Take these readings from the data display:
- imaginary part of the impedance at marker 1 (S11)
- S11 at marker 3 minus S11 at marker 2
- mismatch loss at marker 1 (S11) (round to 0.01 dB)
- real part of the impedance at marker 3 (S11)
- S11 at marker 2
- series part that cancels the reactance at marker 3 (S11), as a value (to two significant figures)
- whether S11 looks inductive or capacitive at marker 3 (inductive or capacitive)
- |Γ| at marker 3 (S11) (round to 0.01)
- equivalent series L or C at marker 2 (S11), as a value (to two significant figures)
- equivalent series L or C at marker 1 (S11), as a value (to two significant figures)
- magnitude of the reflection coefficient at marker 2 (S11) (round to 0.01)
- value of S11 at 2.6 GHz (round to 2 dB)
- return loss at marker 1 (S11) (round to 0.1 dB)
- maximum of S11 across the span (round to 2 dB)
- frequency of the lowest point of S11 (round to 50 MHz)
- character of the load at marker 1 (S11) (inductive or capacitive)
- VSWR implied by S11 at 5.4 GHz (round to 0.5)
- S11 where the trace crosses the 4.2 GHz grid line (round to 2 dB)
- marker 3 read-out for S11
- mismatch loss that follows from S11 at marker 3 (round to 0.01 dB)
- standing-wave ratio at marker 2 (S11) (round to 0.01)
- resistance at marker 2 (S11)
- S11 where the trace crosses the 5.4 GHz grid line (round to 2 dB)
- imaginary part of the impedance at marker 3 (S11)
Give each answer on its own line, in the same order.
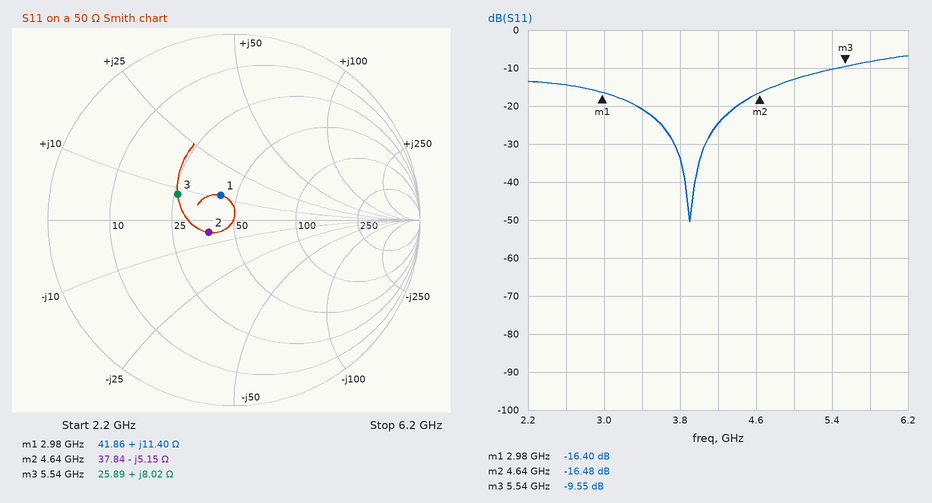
+11.40 Ω
6.93 dB
0.10 dB
25.89 Ω
-16.48 dB
3.6 pF
inductive
0.33
6.7 pF
610 pH
0.15
-14 dB
16.4 dB
-6 dB
3.90 GHz
inductive
2.0
-24 dB
-9.55 dB
0.51 dB
1.35
37.84 Ω
-10 dB
+8.02 Ω
